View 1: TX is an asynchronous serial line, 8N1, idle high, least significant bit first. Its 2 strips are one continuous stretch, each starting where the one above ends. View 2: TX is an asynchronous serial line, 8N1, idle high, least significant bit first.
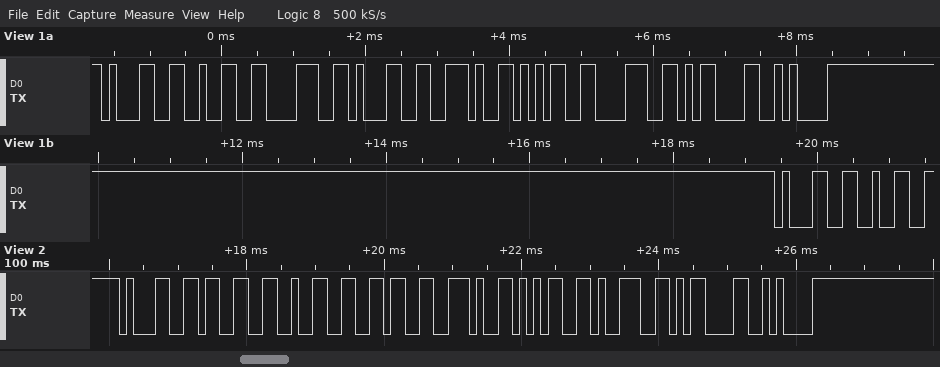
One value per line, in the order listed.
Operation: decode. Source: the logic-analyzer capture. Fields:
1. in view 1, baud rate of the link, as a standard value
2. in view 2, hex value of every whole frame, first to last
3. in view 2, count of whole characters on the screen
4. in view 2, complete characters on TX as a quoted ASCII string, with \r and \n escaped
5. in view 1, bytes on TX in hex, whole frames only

9600 baud
0x31 0x33 0x32 0x36 0x2E 0x35 0x39 0x0D 0x0A
9
"1326.59\r\n"
31 32 38 31 2E 35 38 0D 0A 31 32
